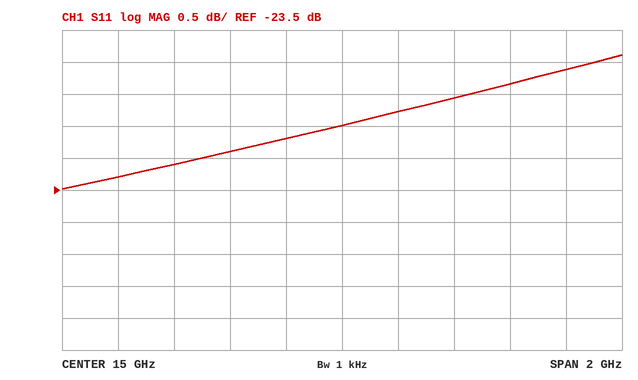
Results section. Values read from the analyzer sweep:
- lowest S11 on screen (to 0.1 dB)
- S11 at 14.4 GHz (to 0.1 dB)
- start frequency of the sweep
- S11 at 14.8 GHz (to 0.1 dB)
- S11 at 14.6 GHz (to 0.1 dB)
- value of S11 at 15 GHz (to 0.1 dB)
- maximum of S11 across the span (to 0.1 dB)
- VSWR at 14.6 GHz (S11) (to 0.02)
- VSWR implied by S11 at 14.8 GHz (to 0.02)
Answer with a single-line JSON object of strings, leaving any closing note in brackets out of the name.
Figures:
{"lowest S11 on screen": "-23.5 dB", "S11 at 14.4 GHz": "-23.1 dB", "start frequency of the sweep": "14 GHz", "S11 at 14.8 GHz": "-22.7 dB", "S11 at 14.6 GHz": "-22.9 dB", "value of S11 at 15 GHz": "-22.5 dB", "maximum of S11 across the span": "-21.4 dB", "VSWR at 14.6 GHz (S11)": "1.16", "VSWR implied by S11 at 14.8 GHz": "1.16"}
